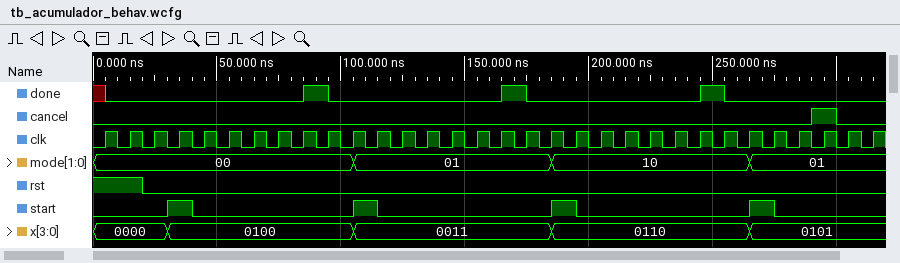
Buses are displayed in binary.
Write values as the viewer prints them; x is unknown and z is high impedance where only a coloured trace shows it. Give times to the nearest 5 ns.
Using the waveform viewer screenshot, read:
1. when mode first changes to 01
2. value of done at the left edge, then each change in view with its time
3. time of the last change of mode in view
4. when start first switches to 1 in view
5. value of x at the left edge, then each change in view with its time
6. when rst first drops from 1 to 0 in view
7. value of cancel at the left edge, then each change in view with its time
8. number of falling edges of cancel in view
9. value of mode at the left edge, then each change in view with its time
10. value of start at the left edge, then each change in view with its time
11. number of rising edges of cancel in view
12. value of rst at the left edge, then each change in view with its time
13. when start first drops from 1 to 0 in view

105 ns
x, 0 at 5 ns, 1 at 85 ns, 0 at 95 ns, 1 at 165 ns, 0 at 175 ns, 1 at 245 ns, 0 at 255 ns
265 ns
30 ns
0000, 0100 at 30 ns, 0011 at 105 ns, 0110 at 185 ns, 0101 at 265 ns
20 ns
0, 1 at 290 ns, 0 at 300 ns
1
00, 01 at 105 ns, 10 at 185 ns, 01 at 265 ns
0, 1 at 30 ns, 0 at 40 ns, 1 at 105 ns, 0 at 115 ns, 1 at 185 ns, 0 at 195 ns, 1 at 265 ns, 0 at 275 ns
1
1, 0 at 20 ns
40 ns
